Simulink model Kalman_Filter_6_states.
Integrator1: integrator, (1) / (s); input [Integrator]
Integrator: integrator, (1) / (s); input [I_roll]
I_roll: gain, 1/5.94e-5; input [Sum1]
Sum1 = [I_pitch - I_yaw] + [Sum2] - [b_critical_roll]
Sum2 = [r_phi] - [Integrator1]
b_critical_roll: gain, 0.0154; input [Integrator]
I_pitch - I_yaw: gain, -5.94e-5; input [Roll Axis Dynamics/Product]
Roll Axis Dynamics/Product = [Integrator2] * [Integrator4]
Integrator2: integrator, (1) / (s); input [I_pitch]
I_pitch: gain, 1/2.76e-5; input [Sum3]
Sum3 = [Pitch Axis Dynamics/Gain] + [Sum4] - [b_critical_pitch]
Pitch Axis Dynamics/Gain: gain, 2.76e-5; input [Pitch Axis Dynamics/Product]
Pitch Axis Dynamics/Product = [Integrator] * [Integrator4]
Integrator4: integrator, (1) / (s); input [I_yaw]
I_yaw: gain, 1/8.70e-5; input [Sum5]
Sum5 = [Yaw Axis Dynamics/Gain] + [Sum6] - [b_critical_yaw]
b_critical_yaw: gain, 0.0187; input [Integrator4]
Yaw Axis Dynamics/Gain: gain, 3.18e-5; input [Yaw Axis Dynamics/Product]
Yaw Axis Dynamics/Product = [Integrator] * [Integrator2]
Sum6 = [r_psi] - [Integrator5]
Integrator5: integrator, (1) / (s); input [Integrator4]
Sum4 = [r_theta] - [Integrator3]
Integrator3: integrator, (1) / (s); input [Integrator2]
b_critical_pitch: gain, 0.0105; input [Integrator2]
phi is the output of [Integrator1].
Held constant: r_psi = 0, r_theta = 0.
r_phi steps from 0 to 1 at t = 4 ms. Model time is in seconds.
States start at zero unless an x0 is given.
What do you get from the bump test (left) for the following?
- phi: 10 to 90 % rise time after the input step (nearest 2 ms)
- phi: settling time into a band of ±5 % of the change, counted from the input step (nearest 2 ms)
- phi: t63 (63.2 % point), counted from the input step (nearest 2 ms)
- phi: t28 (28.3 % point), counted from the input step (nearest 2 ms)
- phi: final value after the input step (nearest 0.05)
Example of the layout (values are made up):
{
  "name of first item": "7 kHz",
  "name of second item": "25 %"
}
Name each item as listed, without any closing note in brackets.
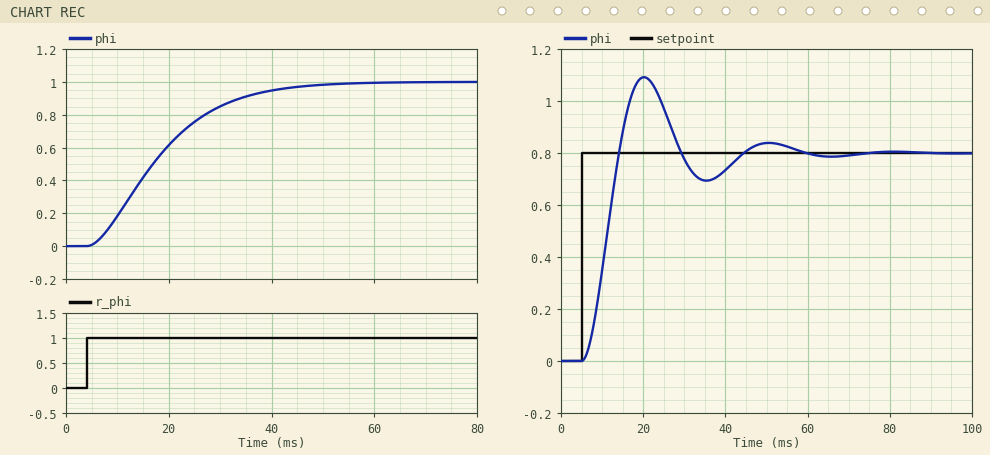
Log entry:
{
  "phi: 10 to 90 % rise time after the input step": "26 ms",
  "phi: settling time into a band of ±5 % of the change, counted from the input step": "36 ms",
  "phi: t63 (63.2 % point), counted from the input step": "16 ms",
  "phi: t28 (28.3 % point), counted from the input step": "8 ms",
  "phi: final value after the input step": "1.00"
}
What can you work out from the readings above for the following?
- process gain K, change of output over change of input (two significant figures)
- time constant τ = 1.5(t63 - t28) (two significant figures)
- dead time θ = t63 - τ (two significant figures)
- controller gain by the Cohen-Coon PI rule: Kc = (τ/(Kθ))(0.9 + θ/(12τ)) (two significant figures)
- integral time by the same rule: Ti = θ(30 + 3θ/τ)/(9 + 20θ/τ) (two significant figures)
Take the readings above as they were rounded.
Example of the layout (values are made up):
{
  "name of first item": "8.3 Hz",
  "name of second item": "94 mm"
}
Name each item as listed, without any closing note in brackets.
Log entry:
{
  "process gain K, change of output over change of input": "1.0",
  "time constant τ = 1.5(t63 - t28)": "12 ms",
  "dead time θ = t63 - τ": "4.0 ms",
  "controller gain by the Cohen-Coon PI rule: Kc = (τ/(Kθ))(0.9 + θ/(12τ))": "2.8",
  "integral time by the same rule: Ti = θ(30 + 3θ/τ)/(9 + 20θ/τ)": "7.9 ms"
}
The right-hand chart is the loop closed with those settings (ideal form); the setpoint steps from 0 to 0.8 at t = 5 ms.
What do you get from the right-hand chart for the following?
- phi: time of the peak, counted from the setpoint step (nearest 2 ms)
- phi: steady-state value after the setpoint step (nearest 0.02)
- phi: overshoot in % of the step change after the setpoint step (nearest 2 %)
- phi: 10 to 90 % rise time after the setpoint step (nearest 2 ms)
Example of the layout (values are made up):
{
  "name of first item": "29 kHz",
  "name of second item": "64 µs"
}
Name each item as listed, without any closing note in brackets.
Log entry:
{
  "phi: time of the peak, counted from the setpoint step": "16 ms",
  "phi: steady-state value after the setpoint step": "0.80",
  "phi: overshoot in % of the step change after the setpoint step": "36 %",
  "phi: 10 to 90 % rise time after the setpoint step": "6 ms"
}
